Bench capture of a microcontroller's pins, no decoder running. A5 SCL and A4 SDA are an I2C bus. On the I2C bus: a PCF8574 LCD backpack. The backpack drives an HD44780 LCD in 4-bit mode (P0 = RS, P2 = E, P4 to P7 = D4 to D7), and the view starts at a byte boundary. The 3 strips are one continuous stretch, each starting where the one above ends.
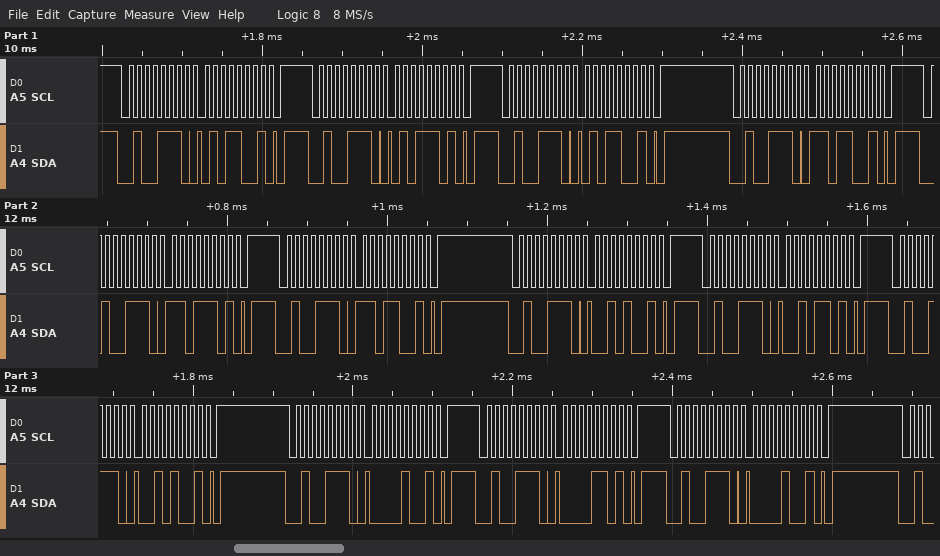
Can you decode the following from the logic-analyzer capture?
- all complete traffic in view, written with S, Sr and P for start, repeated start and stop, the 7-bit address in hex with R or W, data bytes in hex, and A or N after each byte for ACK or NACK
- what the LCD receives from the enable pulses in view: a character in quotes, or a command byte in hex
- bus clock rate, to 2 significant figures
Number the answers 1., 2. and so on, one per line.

1. S 27W A 59 A P S 27W A 5D A P S 27W A 59 A P S 27W A D9 A P S 27W A DD A P S 27W A D9 A P S 27W A 29 A P S 27W A 2D A P S 27W A 29 A P S 27W A 09 A P S 27W A 0D A P S 27W A 09 A P
2. ']' ' '
3. 100 kHz
